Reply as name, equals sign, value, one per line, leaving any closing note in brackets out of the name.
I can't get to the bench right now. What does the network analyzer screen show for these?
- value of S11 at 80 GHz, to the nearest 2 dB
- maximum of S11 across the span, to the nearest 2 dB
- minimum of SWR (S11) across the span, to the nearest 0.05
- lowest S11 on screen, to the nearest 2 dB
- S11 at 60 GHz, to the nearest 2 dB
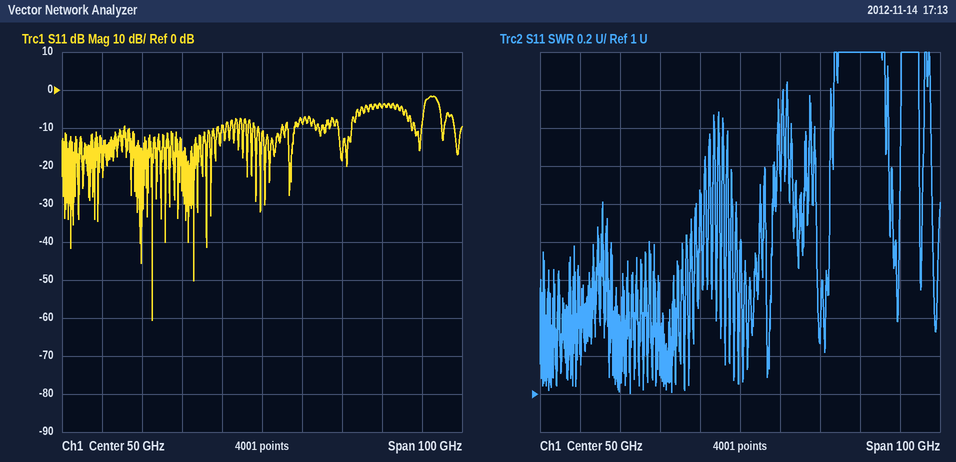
value of S11 at 80 GHz, to the nearest 2 dB = -4 dB
maximum of S11 across the span, to the nearest 2 dB = -2 dB
minimum of SWR (S11) across the span, to the nearest 0.05 = 1.00
lowest S11 on screen, to the nearest 2 dB = -60 dB
S11 at 60 GHz, to the nearest 2 dB = -8 dB
